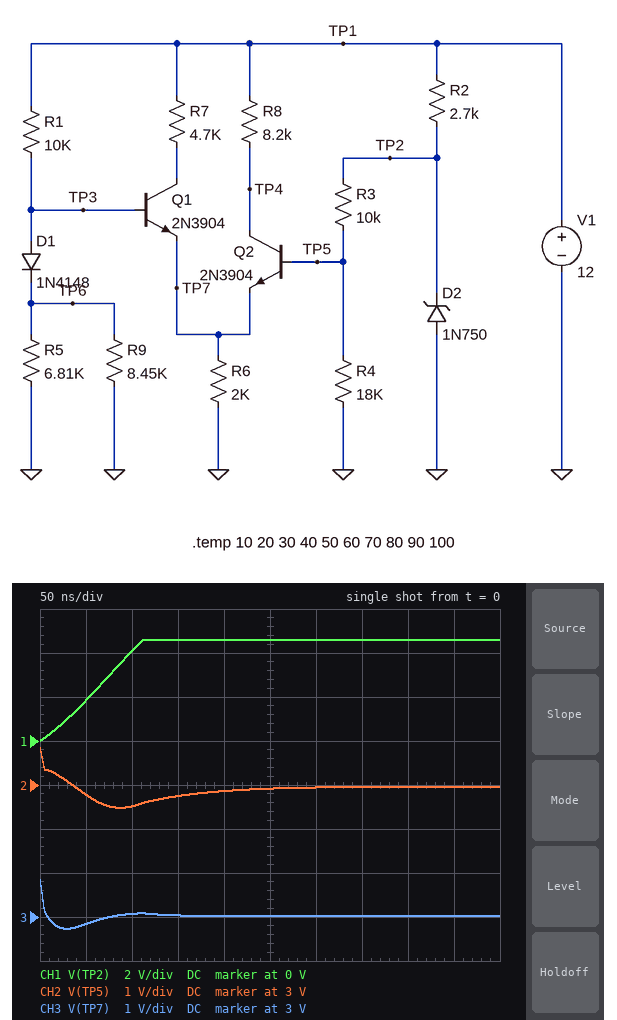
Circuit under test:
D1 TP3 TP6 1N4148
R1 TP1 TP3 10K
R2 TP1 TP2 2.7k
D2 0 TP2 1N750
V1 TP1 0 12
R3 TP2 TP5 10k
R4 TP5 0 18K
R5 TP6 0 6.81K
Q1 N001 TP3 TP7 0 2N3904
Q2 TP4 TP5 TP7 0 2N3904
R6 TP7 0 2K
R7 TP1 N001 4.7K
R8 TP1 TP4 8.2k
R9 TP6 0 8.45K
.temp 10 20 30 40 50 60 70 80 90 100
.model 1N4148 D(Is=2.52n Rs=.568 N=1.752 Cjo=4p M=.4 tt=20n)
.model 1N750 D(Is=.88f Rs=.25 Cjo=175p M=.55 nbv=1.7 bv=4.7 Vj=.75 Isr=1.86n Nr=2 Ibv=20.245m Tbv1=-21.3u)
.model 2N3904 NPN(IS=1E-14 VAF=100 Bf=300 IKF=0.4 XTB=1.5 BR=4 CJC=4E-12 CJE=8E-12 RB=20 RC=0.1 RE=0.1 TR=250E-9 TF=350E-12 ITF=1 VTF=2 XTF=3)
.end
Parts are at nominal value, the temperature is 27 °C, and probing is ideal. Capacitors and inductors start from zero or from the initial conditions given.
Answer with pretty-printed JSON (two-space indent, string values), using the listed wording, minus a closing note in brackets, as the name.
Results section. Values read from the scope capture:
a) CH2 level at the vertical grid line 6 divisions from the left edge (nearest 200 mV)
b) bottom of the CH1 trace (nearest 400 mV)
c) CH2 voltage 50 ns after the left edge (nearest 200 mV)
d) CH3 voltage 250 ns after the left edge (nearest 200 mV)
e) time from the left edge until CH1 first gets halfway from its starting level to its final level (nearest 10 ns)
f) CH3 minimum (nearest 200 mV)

{
  "CH2 level at the vertical grid line 6 divisions from the left edge": "3.0 V",
  "bottom of the CH1 trace": "0 V",
  "CH2 voltage 50 ns after the left edge": "2.8 V",
  "CH3 voltage 250 ns after the left edge": "3.0 V",
  "time from the left edge until CH1 first gets halfway from its starting level to its final level": "60 ns",
  "CH3 minimum": "2.8 V"
}
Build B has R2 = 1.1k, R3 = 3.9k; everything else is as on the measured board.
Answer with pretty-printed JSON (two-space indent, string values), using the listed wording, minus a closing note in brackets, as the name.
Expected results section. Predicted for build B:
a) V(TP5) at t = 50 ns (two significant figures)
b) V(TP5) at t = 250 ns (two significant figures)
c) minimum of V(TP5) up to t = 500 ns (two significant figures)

{
  "V(TP5) at t = 50 ns": "3.4 V",
  "V(TP5) at t = 250 ns": "3.7 V",
  "minimum of V(TP5) up to t = 500 ns": "2.9 V"
}
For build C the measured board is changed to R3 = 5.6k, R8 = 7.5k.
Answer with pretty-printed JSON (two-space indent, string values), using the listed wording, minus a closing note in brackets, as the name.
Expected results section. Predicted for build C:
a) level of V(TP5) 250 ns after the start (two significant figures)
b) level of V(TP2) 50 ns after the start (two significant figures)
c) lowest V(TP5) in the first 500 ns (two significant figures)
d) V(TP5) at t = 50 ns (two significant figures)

{
  "level of V(TP5) 250 ns after the start": "3.5 V",
  "level of V(TP2) 50 ns after the start": "1.9 V",
  "lowest V(TP5) in the first 500 ns": "2.2 V",
  "V(TP5) at t = 50 ns": "2.3 V"
}
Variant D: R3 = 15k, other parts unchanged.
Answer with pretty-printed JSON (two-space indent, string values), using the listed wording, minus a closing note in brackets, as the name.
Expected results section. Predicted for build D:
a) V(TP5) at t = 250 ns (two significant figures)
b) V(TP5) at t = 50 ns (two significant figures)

{
  "V(TP5) at t = 250 ns": "2.5 V",
  "V(TP5) at t = 50 ns": "3.0 V"
}
